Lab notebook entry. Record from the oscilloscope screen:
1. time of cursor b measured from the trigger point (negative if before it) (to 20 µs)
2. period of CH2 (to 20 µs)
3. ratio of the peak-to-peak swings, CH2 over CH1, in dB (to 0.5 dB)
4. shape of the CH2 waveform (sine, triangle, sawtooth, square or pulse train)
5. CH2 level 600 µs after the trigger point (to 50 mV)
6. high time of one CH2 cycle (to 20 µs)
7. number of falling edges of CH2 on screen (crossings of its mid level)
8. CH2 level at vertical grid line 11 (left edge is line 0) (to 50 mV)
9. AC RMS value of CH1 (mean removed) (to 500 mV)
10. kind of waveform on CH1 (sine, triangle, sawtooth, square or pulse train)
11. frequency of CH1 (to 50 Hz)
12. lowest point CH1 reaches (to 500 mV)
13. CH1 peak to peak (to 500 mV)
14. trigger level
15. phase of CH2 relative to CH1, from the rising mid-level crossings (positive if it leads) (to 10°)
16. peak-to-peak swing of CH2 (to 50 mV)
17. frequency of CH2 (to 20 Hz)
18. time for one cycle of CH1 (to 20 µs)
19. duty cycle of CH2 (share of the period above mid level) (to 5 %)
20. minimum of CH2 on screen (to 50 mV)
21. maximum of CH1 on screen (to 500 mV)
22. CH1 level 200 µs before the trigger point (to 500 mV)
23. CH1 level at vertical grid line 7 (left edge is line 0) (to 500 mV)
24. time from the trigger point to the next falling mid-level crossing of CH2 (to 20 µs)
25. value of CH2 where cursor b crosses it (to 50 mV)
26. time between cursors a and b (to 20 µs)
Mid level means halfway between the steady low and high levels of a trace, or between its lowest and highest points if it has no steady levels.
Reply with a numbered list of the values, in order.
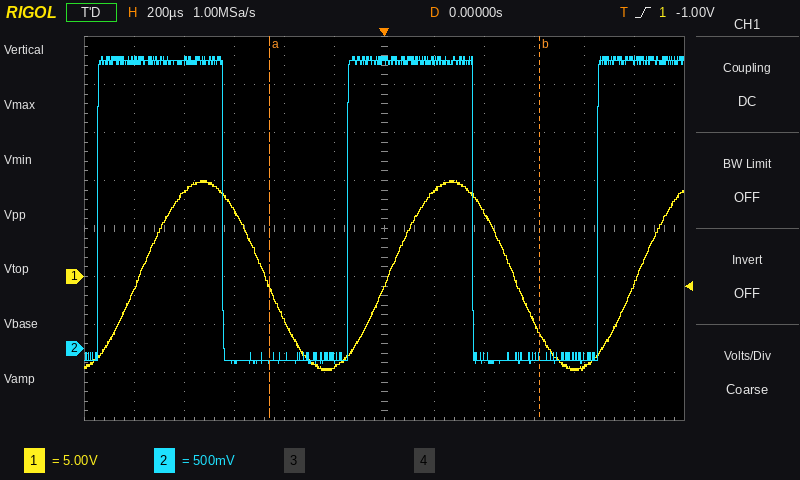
1. +620 µs
2. 1.00 ms
3. -16.0 dB
4. square
5. -100 mV
6. 500 µs
7. 2
8. 3.00 V
9. 7.0 V
10. sine
11. 1.00 kHz
12. -10.0 V
13. 20.0 V
14. -1.00 V
15. +60°
16. 3.20 V
17. 1.00 kHz
18. 1.00 ms
19. 50 %
20. -150 mV
21. 10.0 V
22. -9.5 V
23. 9.0 V
24. 360 µs
25. -100 mV
26. 1.08 ms
